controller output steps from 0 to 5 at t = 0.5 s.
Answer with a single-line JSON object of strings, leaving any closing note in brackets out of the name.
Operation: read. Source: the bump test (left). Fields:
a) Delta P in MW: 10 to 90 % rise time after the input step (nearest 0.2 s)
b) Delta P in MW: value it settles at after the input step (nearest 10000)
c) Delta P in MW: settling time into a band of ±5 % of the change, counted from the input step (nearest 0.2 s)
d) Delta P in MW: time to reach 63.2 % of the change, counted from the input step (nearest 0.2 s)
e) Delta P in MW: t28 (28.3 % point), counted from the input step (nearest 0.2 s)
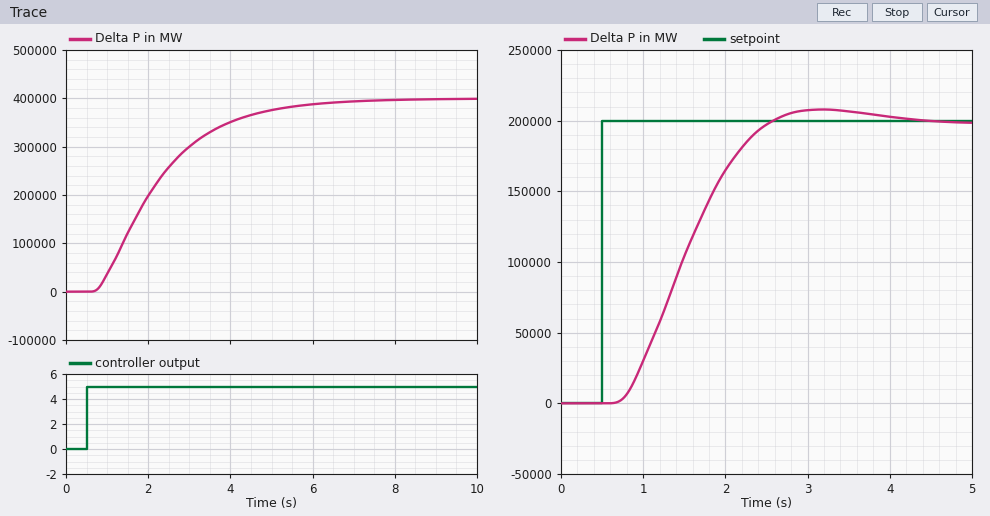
{"Delta P in MW: 10 to 90 % rise time after the input step": "3.2 s", "Delta P in MW: value it settles at after the input step": "400000", "Delta P in MW: settling time into a band of ±5 % of the change, counted from the input step": "4.8 s", "Delta P in MW: time to reach 63.2 % of the change, counted from the input step": "2.0 s", "Delta P in MW: t28 (28.3 % point), counted from the input step": "1.0 s"}
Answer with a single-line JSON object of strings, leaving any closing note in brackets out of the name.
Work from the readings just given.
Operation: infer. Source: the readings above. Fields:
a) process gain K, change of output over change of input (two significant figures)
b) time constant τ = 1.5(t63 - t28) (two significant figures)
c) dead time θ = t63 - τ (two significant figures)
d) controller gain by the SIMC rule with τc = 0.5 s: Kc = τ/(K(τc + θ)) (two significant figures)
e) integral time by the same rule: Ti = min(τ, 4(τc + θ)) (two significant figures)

{"process gain K, change of output over change of input": "80000", "time constant τ = 1.5(t63 - t28)": "1.5 s", "dead time θ = t63 - τ": "0.50 s", "controller gain by the SIMC rule with τc = 0.5 s: Kc = τ/(K(τc + θ))": "0.000019", "integral time by the same rule: Ti = min(τ, 4(τc + θ))": "1.5 s"}
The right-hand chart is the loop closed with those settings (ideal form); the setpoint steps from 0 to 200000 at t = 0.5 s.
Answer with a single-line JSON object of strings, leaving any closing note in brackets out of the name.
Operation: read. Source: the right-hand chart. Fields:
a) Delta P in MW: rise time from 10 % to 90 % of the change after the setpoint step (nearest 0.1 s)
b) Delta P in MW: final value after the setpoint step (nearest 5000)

{"Delta P in MW: rise time from 10 % to 90 % of the change after the setpoint step": "1.3 s", "Delta P in MW: final value after the setpoint step": "200000"}
